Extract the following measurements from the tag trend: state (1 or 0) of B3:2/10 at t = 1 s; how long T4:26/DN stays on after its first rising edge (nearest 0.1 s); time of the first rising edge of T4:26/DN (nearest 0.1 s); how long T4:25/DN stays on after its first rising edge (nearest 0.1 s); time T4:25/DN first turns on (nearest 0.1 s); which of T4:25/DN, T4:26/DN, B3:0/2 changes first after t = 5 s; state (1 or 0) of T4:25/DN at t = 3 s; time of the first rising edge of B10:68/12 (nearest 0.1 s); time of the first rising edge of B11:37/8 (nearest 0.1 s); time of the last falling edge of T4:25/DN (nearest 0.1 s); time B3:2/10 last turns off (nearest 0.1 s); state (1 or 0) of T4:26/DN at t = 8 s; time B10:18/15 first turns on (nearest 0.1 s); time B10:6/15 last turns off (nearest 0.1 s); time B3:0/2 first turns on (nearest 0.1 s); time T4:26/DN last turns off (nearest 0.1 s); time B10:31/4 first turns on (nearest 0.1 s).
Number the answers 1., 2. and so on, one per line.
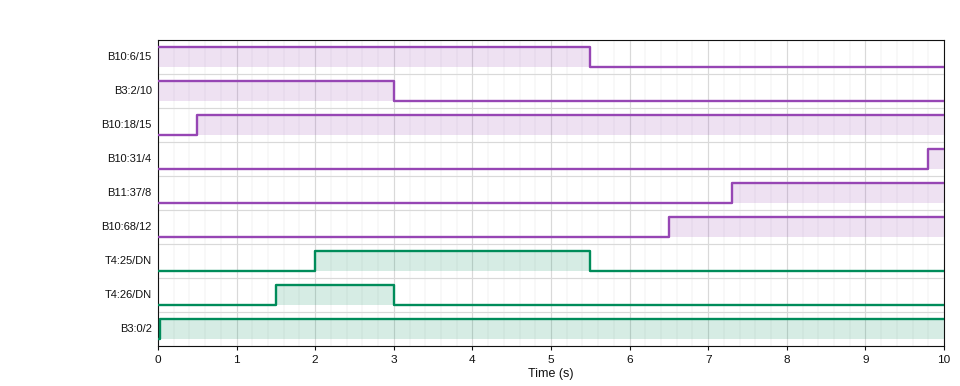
1. 1
2. 1.5 s
3. 1.5 s
4. 3.5 s
5. 2.0 s
6. T4:25/DN
7. 1
8. 6.5 s
9. 7.3 s
10. 5.5 s
11. 3.0 s
12. 0
13. 0.5 s
14. 5.5 s
15. 0.0 s
16. 3.0 s
17. 9.8 s
